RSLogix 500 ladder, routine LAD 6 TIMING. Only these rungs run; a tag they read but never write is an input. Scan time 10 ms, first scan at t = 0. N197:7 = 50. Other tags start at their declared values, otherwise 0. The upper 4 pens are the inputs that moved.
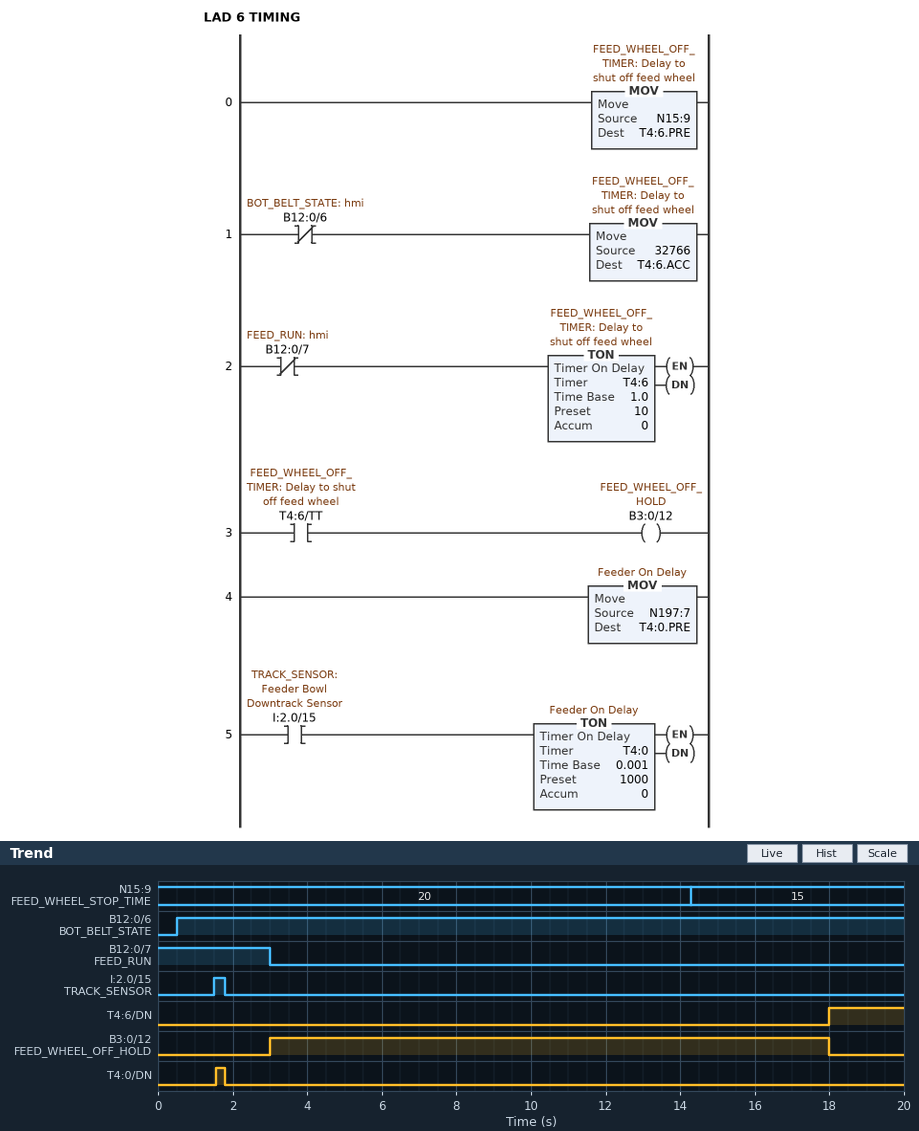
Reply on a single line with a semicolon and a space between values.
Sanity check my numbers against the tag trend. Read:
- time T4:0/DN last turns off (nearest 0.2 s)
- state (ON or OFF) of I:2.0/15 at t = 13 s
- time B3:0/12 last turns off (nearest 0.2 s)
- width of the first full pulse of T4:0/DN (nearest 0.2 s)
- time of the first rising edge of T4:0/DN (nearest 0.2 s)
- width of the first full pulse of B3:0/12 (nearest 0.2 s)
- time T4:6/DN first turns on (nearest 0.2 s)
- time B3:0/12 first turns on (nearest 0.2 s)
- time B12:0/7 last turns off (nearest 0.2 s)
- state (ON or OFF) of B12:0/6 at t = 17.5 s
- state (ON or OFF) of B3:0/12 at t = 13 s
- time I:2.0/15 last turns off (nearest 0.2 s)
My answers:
1.8 s; OFF; 18.0 s; 0.2 s; 1.6 s; 15.0 s; 18.0 s; 3.0 s; 3.0 s; ON; ON; 1.8 s
